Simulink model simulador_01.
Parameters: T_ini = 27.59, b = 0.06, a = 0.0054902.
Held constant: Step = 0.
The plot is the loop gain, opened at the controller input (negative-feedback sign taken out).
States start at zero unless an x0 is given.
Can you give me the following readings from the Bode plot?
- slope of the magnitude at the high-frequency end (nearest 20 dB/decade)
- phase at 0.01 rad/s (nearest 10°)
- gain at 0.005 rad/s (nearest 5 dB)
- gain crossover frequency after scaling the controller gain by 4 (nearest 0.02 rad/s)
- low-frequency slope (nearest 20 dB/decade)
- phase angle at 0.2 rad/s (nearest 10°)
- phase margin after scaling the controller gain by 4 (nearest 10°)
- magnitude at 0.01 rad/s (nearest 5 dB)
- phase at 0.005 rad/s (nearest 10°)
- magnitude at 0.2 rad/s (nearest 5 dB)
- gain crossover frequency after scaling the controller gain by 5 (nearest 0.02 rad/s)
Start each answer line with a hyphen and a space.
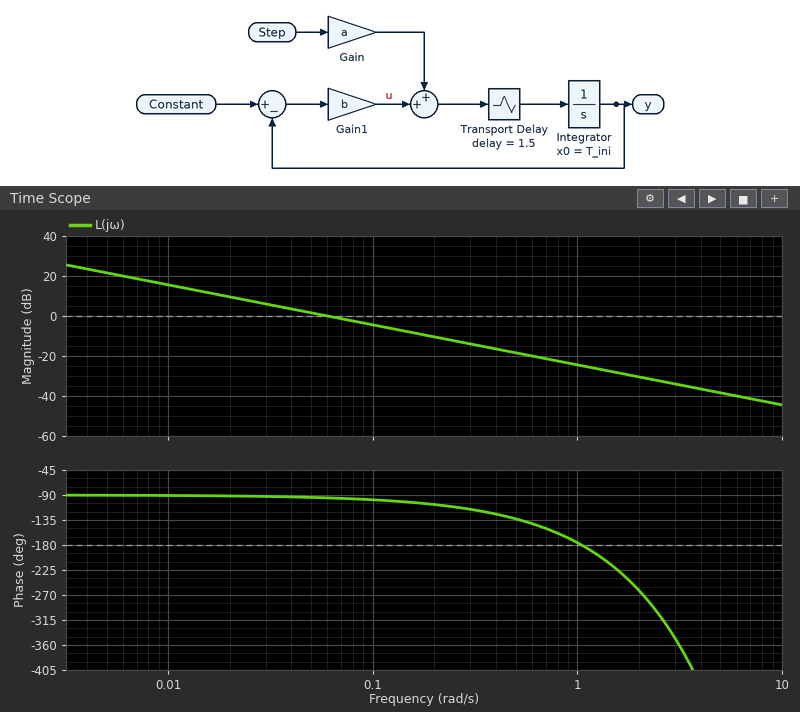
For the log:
- -20 dB/decade
- -90°
- 20 dB
- 0.24 rad/s
- -20 dB/decade
- -110°
- 70°
- 15 dB
- -90°
- -10 dB
- 0.30 rad/s
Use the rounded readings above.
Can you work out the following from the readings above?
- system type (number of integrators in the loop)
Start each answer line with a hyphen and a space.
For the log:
- 1
